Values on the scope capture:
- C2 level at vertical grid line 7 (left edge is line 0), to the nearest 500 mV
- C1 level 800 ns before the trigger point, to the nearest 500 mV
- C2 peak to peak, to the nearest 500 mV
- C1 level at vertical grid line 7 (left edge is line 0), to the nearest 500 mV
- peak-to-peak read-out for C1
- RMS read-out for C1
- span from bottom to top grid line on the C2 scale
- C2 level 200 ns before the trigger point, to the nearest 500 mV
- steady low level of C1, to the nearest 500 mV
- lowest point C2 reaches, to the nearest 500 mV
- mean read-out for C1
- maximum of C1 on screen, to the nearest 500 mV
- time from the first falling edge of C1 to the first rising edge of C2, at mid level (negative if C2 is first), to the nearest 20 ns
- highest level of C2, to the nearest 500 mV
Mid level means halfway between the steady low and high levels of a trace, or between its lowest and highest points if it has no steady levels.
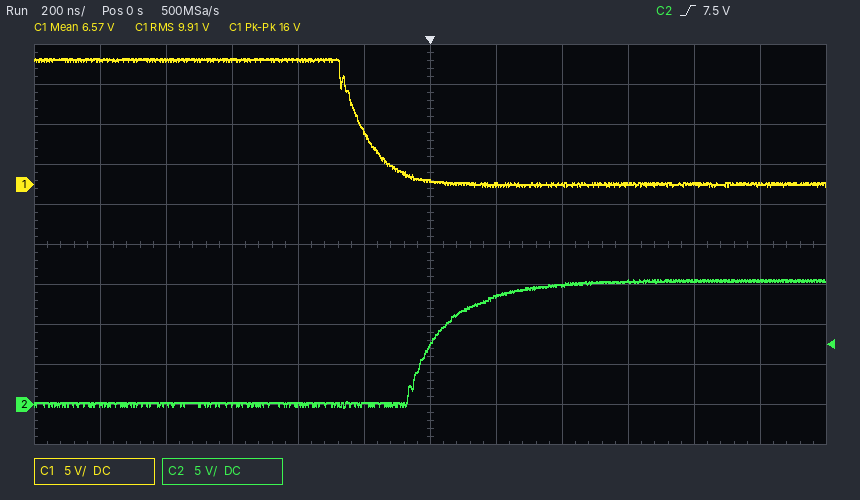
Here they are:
13.5 V
15.5 V
16.0 V
0.0 V
16 V
9.91 V
50 V
0.0 V
0.0 V
-500 mV
6.57 V
16.0 V
+220 ns
15.5 V
